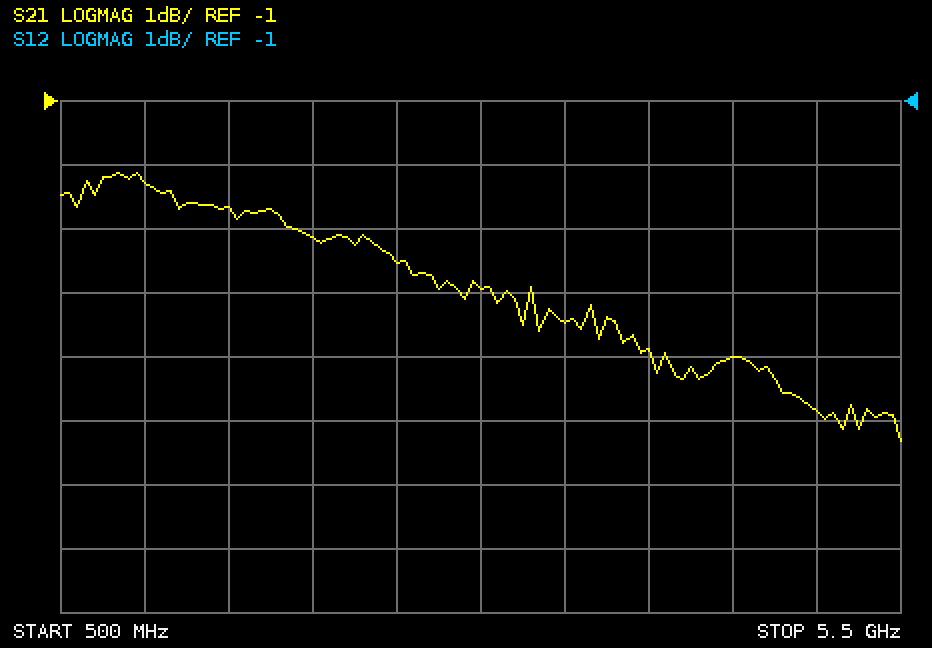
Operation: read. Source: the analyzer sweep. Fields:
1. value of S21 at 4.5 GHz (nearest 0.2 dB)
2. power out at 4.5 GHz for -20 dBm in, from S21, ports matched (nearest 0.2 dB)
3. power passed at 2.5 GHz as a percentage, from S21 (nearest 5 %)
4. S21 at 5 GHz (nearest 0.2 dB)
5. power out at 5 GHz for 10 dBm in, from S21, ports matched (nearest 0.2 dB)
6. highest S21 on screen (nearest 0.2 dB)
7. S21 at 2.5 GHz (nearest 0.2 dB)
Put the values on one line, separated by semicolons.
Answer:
-5.0 dB; -25.0 dBm; 45 %; -5.8 dB; 4.2 dBm; -2.2 dB; -3.6 dB
